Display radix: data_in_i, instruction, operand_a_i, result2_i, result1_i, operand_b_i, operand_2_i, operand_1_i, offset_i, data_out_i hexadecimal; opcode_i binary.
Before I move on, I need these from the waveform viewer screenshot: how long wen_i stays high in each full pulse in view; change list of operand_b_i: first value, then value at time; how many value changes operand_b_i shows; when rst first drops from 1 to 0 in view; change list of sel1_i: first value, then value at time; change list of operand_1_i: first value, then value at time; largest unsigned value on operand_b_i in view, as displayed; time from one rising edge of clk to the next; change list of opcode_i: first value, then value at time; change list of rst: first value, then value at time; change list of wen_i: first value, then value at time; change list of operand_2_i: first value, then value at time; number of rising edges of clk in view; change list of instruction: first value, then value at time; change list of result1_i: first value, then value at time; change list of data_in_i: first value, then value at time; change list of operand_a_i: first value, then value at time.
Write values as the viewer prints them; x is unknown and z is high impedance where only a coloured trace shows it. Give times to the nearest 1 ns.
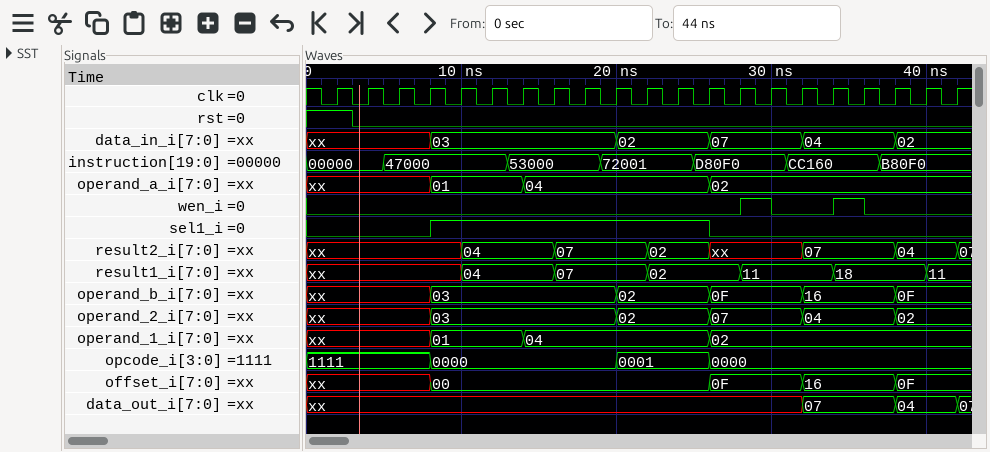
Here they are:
2 ns, 2 ns
xx, 03 at 8 ns, 02 at 20 ns, 0F at 26 ns, 16 at 32 ns, 0F at 38 ns
5
3 ns
0, 1 at 8 ns, 0 at 26 ns
xx, 01 at 8 ns, 04 at 14 ns, 02 at 26 ns
16
2 ns
1111, 0000 at 8 ns, 0001 at 20 ns, 0000 at 26 ns
1, 0 at 3 ns
0, 1 at 28 ns, 0 at 30 ns, 1 at 34 ns, 0 at 36 ns
xx, 03 at 8 ns, 02 at 20 ns, 07 at 26 ns, 04 at 32 ns, 02 at 38 ns
21
00000, 47000 at 5 ns, 53000 at 13 ns, 72001 at 19 ns, D80F0 at 25 ns, CC160 at 31 ns, B80F0 at 37 ns
xx, 04 at 10 ns, 07 at 16 ns, 02 at 22 ns, 11 at 28 ns, 18 at 34 ns, 11 at 40 ns
xx, 03 at 8 ns, 02 at 20 ns, 07 at 26 ns, 04 at 32 ns, 02 at 38 ns
xx, 01 at 8 ns, 04 at 14 ns, 02 at 26 ns
